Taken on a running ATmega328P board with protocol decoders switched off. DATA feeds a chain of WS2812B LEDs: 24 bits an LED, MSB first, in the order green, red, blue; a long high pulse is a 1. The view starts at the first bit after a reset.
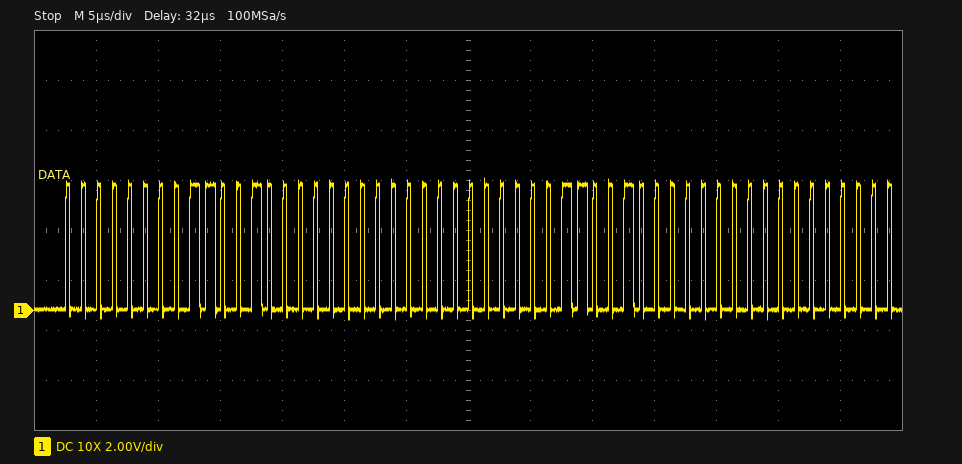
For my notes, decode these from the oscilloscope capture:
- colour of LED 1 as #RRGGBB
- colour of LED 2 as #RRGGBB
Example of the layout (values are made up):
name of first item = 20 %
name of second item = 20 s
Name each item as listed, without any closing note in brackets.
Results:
colour of LED 1 as #RRGGBB = #C80000
colour of LED 2 as #RRGGBB = #C80000
